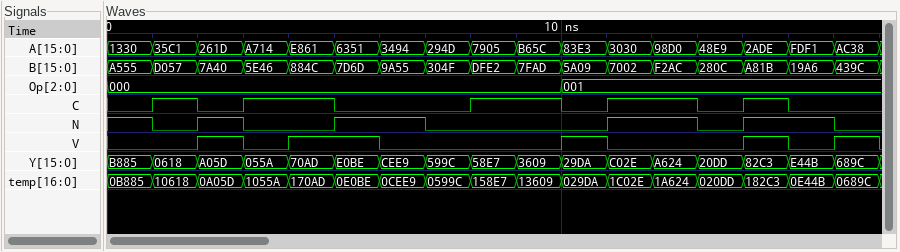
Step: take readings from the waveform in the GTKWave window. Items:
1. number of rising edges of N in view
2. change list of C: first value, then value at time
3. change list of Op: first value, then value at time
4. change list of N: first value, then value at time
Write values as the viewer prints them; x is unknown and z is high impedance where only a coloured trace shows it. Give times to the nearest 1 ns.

4
0, 1 at 1 ns, 0 at 2 ns, 1 at 3 ns, 0 at 5 ns, 1 at 8 ns, 0 at 10 ns, 1 at 11 ns, 0 at 13 ns, 1 at 14 ns, 0 at 15 ns
000, 001 at 10 ns
1, 0 at 1 ns, 1 at 2 ns, 0 at 3 ns, 1 at 5 ns, 0 at 7 ns, 1 at 11 ns, 0 at 13 ns, 1 at 14 ns, 0 at 16 ns
